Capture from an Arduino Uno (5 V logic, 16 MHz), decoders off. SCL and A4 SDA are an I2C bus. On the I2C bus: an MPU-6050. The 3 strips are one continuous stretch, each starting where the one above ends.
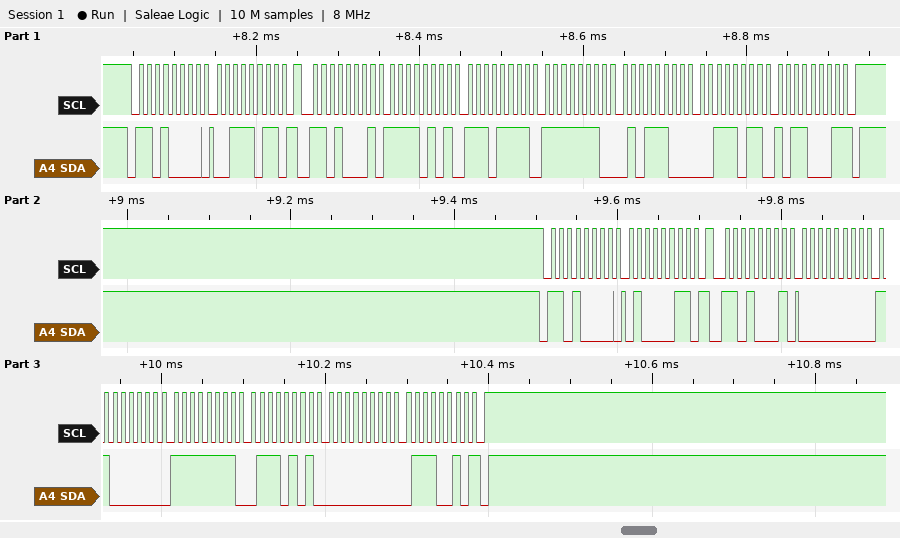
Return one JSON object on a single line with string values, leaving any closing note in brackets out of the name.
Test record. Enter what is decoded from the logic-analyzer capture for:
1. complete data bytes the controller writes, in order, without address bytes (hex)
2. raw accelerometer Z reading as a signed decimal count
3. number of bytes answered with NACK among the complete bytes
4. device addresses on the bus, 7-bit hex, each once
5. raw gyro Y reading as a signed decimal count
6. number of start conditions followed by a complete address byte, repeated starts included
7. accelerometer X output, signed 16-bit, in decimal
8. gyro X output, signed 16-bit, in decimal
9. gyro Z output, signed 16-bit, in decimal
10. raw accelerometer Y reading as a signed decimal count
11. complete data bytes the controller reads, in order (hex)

{"complete data bytes the controller writes, in order, without address bytes": "3B 43", "raw accelerometer Z reading as a signed decimal count": "15281", "number of bytes answered with NACK among the complete bytes": "2", "device addresses on the bus, 7-bit hex, each once": "0x68", "raw gyro Y reading as a signed decimal count": "-139", "number of start conditions followed by a complete address byte, repeated starts included": "4", "accelerometer X output, signed 16-bit, in decimal": "-2577", "gyro X output, signed 16-bit, in decimal": "192", "gyro Z output, signed 16-bit, in decimal": "114", "raw accelerometer Y reading as a signed decimal count": "-420", "complete data bytes the controller reads, in order": "F5 EF FE 5C 3B B1 00 C0 FF 75 00 72"}
